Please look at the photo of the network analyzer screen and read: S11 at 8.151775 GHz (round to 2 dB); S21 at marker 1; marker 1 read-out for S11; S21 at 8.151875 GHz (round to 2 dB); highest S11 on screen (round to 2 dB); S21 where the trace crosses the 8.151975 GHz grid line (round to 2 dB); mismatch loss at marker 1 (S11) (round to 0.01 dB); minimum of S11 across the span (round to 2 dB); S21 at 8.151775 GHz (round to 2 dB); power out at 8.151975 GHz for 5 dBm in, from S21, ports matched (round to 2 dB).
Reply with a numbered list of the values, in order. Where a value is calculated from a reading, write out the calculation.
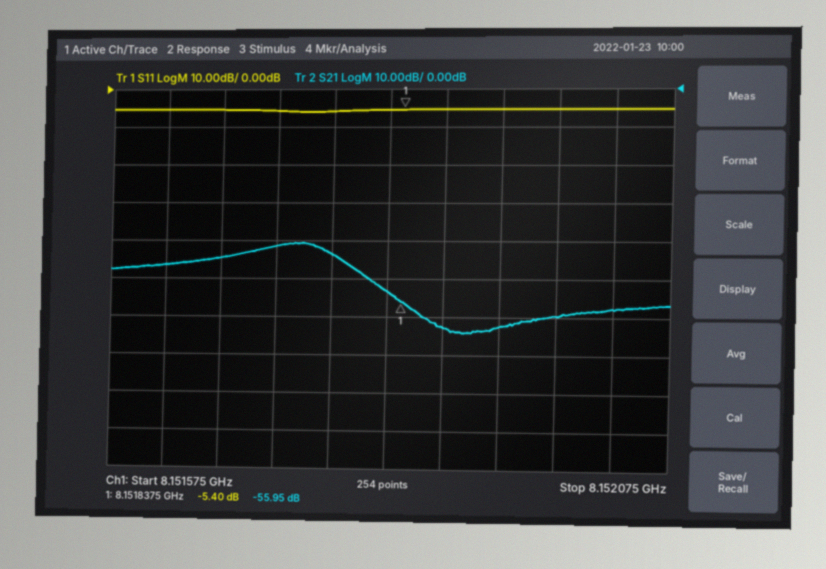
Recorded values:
1. -6 dB
2. -55.95 dB
3. -5.40 dB
4. -62 dB
5. -6 dB
6. -60 dB
7. −10 log10(1 − 10^(-5.4/10)) ≈ 1.48 dB
8. -6 dB
9. -44 dB
10. 5 dBm + (-60 dB) = -54 dBm
